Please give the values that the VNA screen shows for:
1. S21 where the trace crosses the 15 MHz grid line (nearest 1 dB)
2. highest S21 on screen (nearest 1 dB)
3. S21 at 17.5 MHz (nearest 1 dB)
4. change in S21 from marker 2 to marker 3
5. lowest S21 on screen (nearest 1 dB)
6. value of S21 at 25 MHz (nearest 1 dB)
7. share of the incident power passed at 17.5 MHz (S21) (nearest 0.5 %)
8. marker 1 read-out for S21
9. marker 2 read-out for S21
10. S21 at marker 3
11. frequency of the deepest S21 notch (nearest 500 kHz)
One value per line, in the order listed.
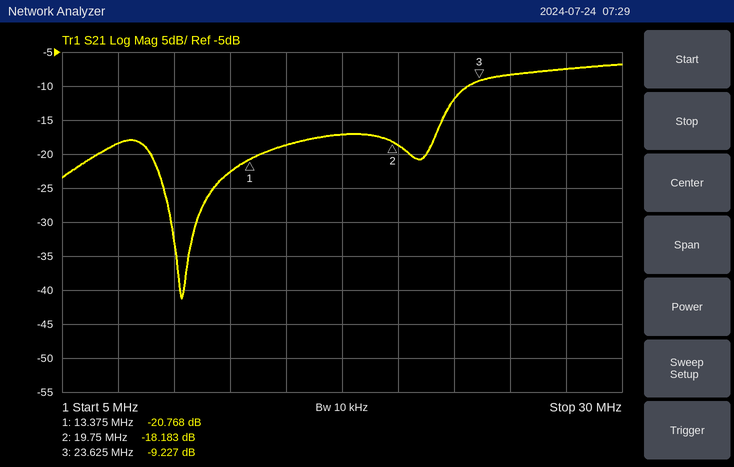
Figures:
-19 dB
-7 dB
-17 dB
8.956 dB
-41 dB
-8 dB
2.0 %
-20.768 dB
-18.183 dB
-9.227 dB
10.5 MHz
